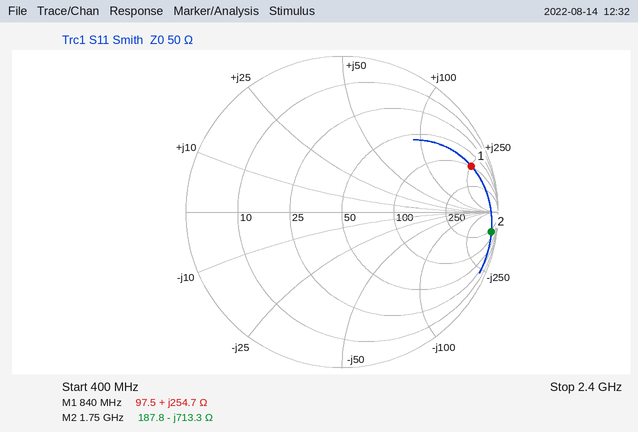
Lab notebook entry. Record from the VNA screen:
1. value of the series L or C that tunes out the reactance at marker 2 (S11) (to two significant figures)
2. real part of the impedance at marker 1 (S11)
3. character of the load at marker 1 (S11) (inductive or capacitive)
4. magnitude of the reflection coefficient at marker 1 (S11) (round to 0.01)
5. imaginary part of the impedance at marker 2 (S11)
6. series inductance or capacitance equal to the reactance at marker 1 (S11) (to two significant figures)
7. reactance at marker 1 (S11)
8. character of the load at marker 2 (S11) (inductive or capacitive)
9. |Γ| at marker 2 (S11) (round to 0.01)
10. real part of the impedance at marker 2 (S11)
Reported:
65 nH
97.5 Ω
inductive
0.88
-713.3 Ω
48 nH
+254.7 Ω
capacitive
0.97
187.8 Ω
